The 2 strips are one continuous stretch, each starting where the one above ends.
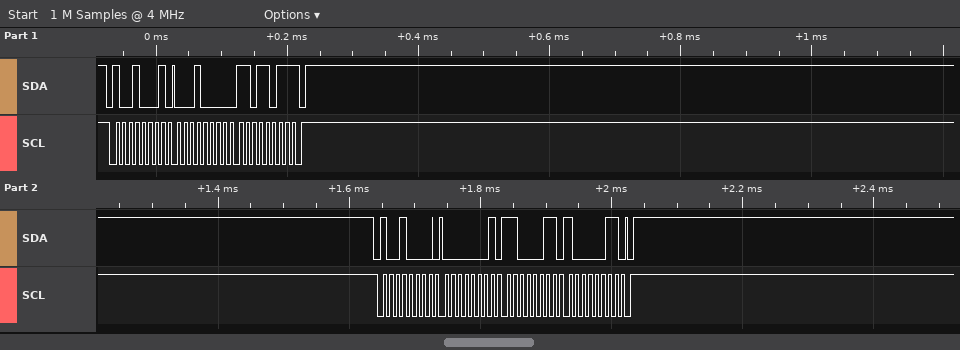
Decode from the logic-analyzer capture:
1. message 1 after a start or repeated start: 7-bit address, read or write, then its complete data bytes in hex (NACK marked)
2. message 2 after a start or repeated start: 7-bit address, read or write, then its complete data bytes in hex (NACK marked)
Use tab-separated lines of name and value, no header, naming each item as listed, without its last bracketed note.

message 1 after a start or repeated start: 7-bit address, read or write, then its complete data bytes in hex	0x48 read: 10 DB NACK
message 2 after a start or repeated start: 7-bit address, read or write, then its complete data bytes in hex	0x48 write: 01 C3 83
